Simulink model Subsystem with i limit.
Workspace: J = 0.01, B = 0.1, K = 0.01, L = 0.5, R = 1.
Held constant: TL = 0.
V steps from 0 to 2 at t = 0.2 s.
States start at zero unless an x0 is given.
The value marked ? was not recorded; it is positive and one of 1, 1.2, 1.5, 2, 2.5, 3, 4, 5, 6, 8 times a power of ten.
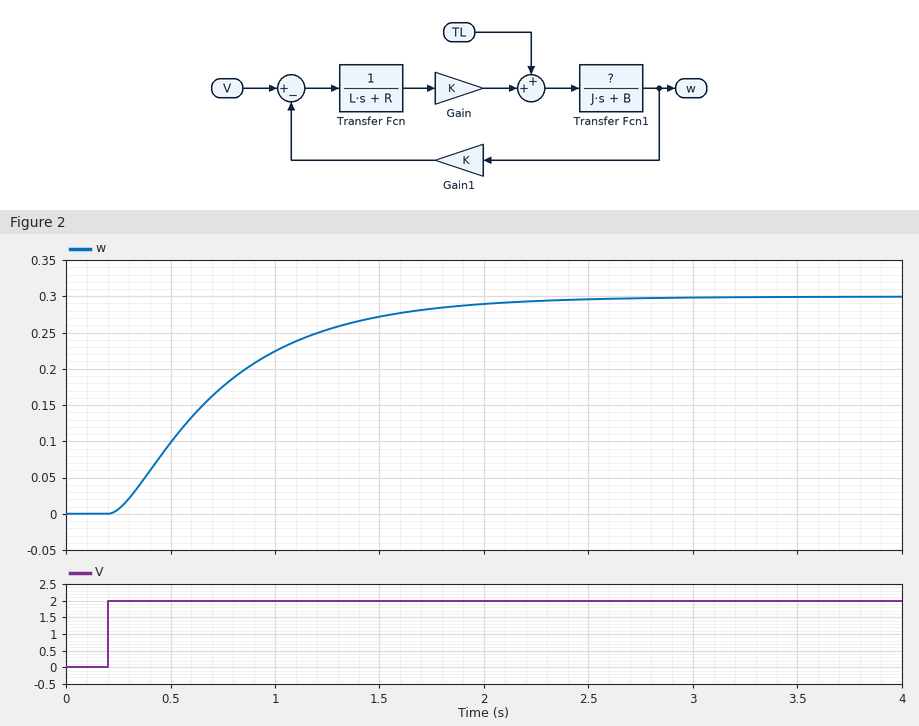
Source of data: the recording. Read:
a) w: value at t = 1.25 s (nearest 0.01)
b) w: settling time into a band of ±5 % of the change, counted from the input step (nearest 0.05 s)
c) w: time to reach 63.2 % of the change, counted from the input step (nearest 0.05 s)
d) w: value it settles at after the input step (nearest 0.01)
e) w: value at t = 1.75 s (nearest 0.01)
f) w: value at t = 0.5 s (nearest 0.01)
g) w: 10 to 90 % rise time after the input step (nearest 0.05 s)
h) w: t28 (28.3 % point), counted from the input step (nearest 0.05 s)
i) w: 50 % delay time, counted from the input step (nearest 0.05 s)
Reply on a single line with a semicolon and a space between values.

0.25; 1.60 s; 0.60 s; 0.30; 0.28; 0.10; 1.15 s; 0.25 s; 0.45 s
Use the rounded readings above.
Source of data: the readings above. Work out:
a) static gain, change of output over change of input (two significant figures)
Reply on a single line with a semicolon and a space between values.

0.15
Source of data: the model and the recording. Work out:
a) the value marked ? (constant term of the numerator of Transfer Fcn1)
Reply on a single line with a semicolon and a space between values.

1.5
